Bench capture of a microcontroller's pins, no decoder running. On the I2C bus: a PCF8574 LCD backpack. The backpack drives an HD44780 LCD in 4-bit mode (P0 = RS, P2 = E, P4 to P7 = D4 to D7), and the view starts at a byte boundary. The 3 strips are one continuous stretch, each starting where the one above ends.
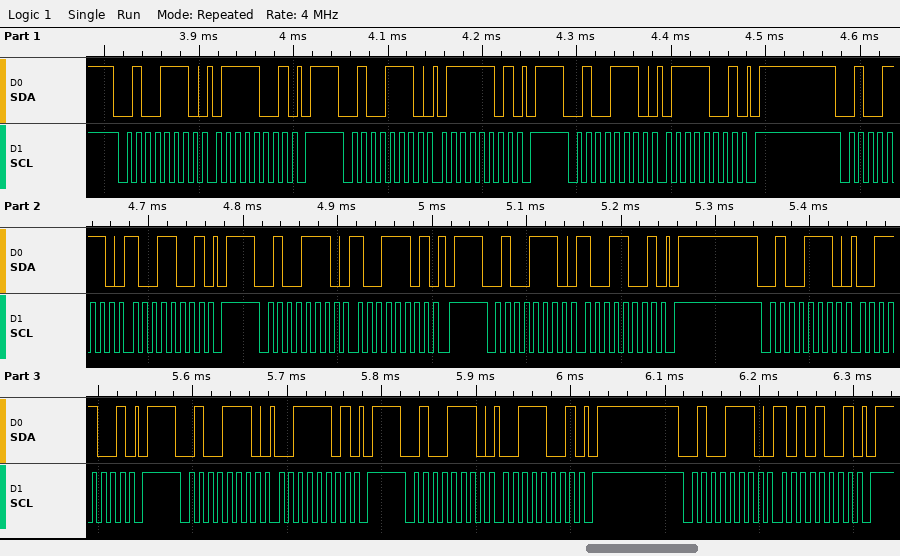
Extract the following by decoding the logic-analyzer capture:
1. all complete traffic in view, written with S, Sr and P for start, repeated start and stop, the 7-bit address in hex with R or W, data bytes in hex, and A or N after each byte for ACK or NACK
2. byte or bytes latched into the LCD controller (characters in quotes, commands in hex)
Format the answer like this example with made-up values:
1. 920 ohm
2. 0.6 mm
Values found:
1. S 27W A 79 A P S 27W A 7D A P S 27W A 79 A P S 27W A 99 A P S 27W A 9D A P S 27W A 99 A P S 27W A 39 A P S 27W A 3D A P S 27W A 39 A P S 27W A A9 A P
2. 'y'
